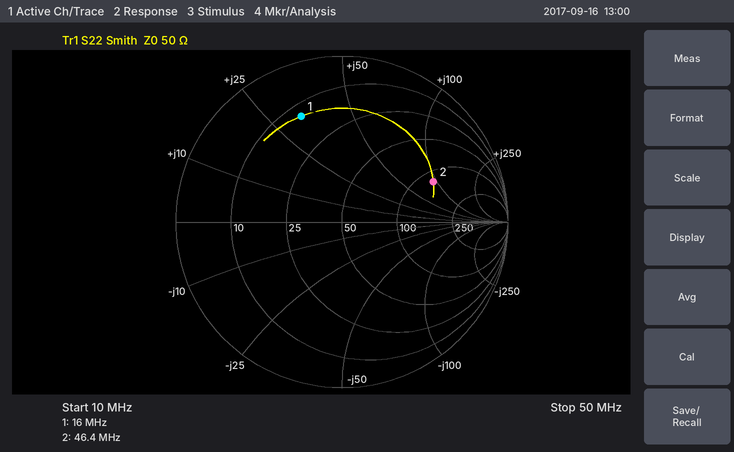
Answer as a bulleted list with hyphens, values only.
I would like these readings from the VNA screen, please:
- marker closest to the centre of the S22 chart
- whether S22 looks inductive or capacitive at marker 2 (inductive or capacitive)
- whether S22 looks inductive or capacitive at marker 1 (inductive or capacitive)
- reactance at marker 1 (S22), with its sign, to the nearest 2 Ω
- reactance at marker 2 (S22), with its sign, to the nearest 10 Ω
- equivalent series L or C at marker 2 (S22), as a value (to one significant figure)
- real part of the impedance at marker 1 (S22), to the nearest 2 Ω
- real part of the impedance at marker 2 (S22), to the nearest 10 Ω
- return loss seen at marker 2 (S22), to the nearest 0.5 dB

- marker 2
- inductive
- inductive
- +32 Ω
- +90 Ω
- 300 nH
- 14 Ω
- 120 Ω
- 4.5 dB
